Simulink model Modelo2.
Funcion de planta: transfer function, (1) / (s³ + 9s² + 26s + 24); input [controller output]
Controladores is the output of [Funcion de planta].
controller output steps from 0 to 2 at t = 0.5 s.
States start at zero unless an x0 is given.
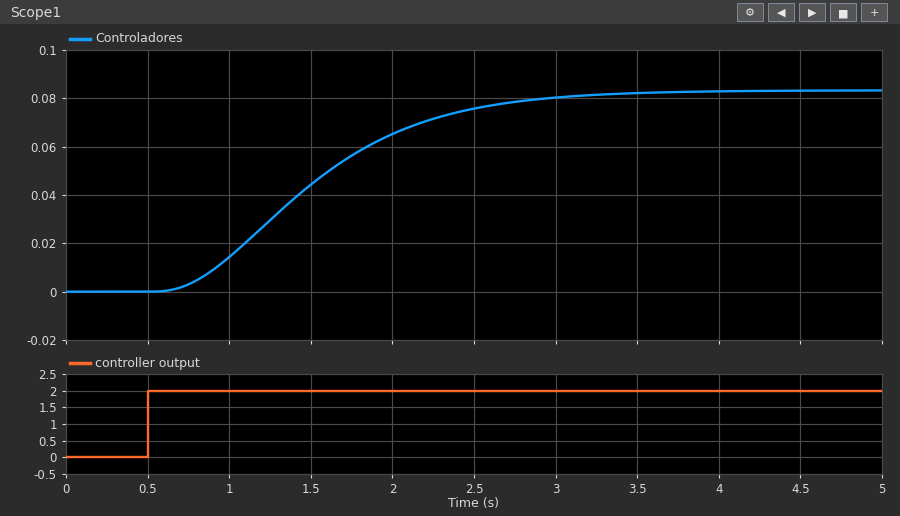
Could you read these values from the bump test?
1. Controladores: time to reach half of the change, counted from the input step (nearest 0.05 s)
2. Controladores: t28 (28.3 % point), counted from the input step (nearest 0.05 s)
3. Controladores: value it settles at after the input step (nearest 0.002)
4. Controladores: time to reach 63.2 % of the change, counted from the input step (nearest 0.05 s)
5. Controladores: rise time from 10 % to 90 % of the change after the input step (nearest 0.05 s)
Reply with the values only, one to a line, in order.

0.95 s
0.65 s
0.084
1.15 s
1.55 s
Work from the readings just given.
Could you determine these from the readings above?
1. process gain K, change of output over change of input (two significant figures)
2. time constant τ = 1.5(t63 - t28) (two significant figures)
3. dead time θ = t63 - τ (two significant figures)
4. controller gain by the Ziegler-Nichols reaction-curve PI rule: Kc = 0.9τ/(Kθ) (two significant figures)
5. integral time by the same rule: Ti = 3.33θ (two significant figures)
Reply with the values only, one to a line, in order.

0.042
0.75 s
0.40 s
40
1.3 s
